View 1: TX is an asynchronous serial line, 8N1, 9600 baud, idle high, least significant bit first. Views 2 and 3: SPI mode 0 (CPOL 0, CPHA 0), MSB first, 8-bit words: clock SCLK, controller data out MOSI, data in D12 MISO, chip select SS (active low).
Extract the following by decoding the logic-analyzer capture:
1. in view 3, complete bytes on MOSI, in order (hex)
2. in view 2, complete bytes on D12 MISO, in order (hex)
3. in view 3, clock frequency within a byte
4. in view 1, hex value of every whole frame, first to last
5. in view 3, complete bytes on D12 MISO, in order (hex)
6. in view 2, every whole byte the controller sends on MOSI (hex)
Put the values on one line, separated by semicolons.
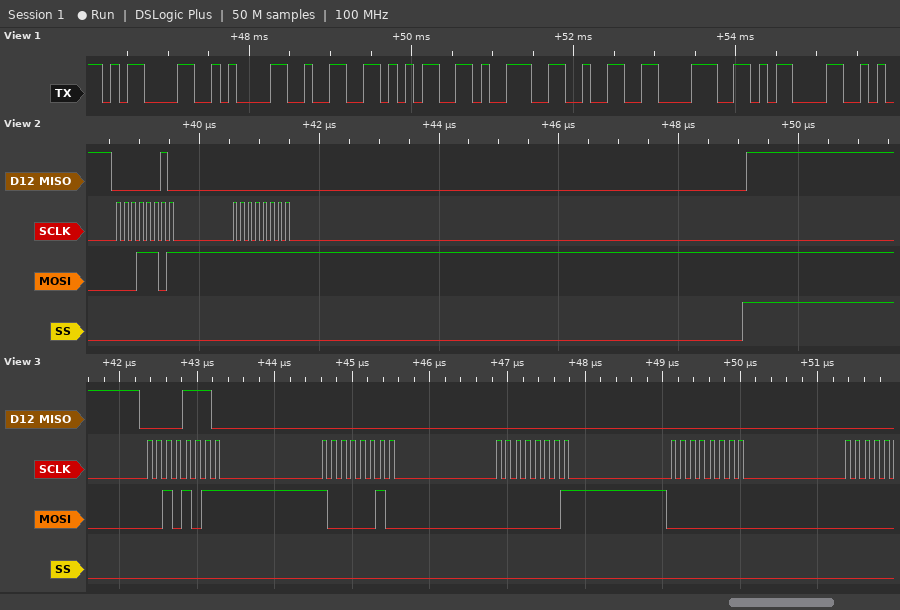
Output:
0x2B 0x82 0x01 0x00; 0x02 0x00; 8 MHz; 0x0D 0x0A 0x32 0x35 0x39 0x32 0x38 0x0D; 0x0E 0x00 0x00 0x00; 0x1D 0xFF
